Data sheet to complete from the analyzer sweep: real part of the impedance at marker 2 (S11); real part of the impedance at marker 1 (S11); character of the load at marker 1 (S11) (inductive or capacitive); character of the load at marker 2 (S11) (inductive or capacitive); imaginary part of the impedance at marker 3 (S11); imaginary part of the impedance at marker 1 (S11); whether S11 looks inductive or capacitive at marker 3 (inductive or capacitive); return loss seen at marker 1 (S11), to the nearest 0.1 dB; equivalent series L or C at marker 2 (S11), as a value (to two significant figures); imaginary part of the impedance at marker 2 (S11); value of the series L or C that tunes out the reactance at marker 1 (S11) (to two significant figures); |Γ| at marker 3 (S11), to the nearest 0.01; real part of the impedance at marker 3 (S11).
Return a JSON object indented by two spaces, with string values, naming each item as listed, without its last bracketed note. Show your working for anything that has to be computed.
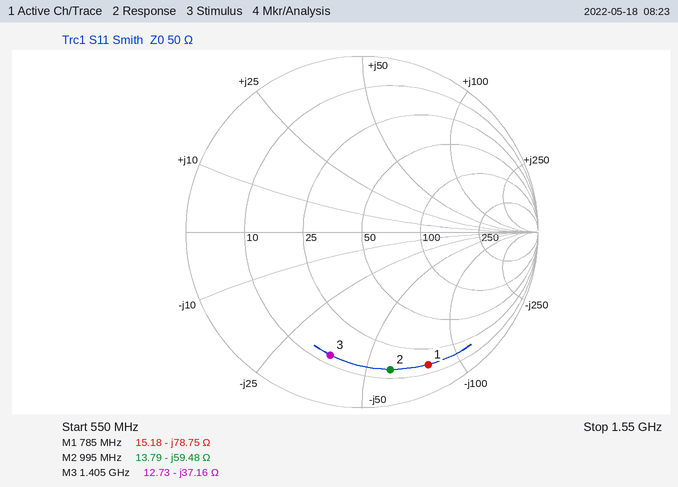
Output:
{
  "real part of the impedance at marker 2": "13.79 Ω",
  "real part of the impedance at marker 1": "15.18 Ω",
  "character of the load at marker 1 (S11)": "capacitive",
  "character of the load at marker 2 (S11)": "capacitive",
  "imaginary part of the impedance at marker 3": "-37.16 Ω",
  "imaginary part of the impedance at marker 1": "-78.75 Ω",
  "whether S11 looks inductive or capacitive at marker 3": "capacitive",
  "return loss seen at marker 1 (S11), to the nearest 0.1 dB": "1.5 dB",
  "equivalent series L or C at marker 2 (S11), as a value": "C = 1/(2π × 995 MHz × 59.48 Ω) ≈ 2.7 pF",
  "imaginary part of the impedance at marker 2": "-59.48 Ω",
  "value of the series L or C that tunes out the reactance at marker 1 (S11)": "L = 78.75 Ω/(2π × 785 MHz) ≈ 16 nH",
  "|Γ| at marker 3 (S11), to the nearest 0.01": "0.72",
  "real part of the impedance at marker 3": "12.73 Ω"
}
